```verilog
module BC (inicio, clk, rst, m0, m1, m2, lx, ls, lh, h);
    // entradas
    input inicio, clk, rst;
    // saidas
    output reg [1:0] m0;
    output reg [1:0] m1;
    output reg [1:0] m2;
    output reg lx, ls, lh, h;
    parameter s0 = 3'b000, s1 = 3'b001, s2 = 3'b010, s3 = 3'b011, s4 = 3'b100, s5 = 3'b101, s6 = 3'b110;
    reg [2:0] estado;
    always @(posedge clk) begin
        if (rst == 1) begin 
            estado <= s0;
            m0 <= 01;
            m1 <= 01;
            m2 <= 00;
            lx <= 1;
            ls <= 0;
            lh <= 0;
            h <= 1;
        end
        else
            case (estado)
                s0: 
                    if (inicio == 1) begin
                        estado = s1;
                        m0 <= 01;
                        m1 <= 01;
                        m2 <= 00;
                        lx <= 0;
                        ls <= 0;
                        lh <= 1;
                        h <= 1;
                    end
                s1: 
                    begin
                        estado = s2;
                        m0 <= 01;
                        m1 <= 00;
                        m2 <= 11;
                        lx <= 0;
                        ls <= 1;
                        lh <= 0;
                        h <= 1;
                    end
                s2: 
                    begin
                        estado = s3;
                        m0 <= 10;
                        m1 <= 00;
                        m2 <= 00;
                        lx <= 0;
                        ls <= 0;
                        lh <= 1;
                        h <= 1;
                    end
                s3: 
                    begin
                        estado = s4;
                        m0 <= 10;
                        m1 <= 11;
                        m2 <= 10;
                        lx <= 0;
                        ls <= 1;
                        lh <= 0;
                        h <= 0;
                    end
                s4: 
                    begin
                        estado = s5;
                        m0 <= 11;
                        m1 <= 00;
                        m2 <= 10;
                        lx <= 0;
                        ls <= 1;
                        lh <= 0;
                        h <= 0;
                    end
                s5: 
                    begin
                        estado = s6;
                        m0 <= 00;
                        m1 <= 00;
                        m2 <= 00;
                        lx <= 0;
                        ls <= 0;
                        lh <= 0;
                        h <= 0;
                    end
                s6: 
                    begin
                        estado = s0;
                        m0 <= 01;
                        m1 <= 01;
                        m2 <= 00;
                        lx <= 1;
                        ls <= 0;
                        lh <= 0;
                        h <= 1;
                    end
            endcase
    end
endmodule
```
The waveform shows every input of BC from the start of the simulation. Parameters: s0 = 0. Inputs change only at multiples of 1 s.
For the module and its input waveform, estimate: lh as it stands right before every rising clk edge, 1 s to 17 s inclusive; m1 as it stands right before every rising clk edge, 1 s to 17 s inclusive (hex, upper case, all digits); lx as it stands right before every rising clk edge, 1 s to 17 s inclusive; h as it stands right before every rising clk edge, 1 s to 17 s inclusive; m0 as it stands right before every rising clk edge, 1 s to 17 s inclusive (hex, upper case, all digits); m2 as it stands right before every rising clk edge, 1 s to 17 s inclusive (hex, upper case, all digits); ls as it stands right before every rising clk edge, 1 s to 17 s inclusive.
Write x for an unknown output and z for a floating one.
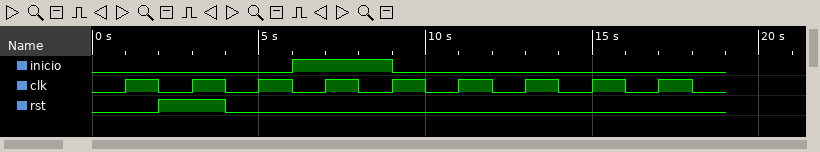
x x 0 0 1 0 1 0 0
x, x, 1, 1, 1, 0, 0, 3, 0
x x 1 1 0 0 0 0 0
x x 1 1 1 1 1 0 0
x, x, 1, 1, 1, 1, 2, 2, 3
x, x, 0, 0, 0, 3, 0, 2, 2
x x 0 0 0 1 0 1 1
